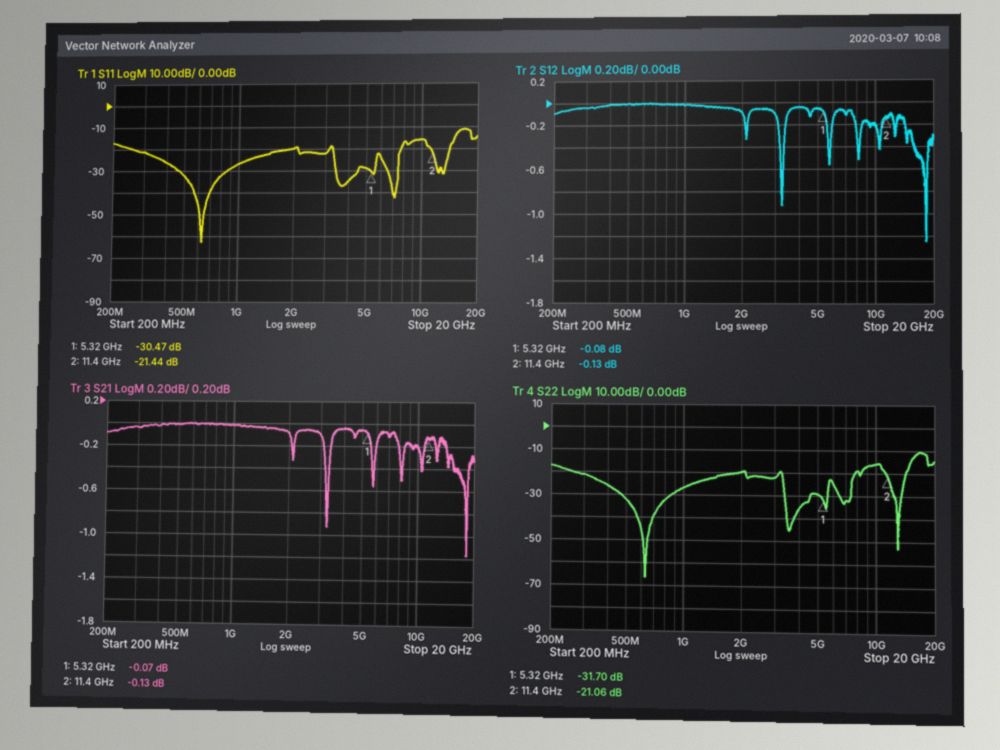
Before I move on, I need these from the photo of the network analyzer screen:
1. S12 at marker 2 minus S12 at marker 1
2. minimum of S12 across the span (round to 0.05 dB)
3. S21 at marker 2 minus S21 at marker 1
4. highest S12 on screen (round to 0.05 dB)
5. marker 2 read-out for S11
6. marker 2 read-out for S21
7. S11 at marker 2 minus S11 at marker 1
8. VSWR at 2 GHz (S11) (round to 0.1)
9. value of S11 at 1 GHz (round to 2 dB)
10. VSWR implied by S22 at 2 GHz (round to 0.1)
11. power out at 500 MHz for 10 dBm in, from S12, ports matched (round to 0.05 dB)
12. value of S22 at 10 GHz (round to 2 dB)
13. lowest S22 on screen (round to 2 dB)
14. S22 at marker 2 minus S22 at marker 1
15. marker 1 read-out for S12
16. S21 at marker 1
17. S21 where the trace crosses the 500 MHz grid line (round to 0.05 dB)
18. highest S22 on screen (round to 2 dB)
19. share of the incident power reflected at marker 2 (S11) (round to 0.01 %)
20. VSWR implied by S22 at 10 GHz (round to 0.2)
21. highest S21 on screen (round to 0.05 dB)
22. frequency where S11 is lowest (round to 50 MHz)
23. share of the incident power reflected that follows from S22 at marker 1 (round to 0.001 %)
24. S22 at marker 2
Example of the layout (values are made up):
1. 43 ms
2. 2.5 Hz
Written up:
1. -0.05 dB
2. -1.25 dB
3. -0.06 dB
4. 0.00 dB
5. -21.44 dB
6. -0.13 dB
7. 9.03 dB
8. 1.2
9. -26 dB
10. 1.2
11. 10.00 dBm
12. -16 dB
13. -66 dB
14. 10.64 dB
15. -0.08 dB
16. -0.07 dB
17. 0.00 dB
18. -10 dB
19. 0.72 %
20. 1.4
21. 0.00 dB
22. 650 MHz
23. 0.068 %
24. -21.06 dB
